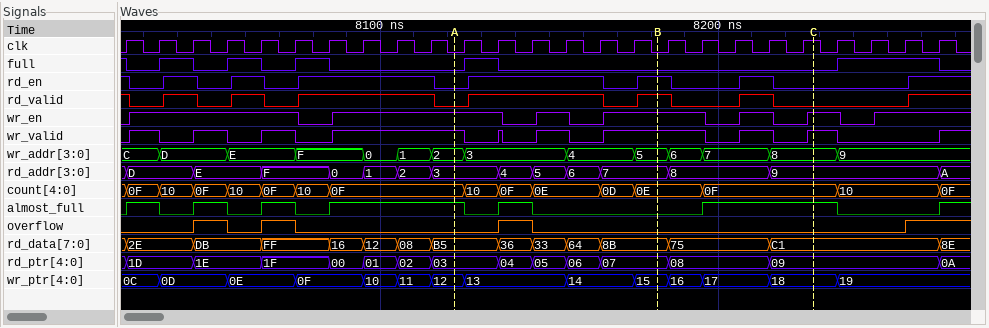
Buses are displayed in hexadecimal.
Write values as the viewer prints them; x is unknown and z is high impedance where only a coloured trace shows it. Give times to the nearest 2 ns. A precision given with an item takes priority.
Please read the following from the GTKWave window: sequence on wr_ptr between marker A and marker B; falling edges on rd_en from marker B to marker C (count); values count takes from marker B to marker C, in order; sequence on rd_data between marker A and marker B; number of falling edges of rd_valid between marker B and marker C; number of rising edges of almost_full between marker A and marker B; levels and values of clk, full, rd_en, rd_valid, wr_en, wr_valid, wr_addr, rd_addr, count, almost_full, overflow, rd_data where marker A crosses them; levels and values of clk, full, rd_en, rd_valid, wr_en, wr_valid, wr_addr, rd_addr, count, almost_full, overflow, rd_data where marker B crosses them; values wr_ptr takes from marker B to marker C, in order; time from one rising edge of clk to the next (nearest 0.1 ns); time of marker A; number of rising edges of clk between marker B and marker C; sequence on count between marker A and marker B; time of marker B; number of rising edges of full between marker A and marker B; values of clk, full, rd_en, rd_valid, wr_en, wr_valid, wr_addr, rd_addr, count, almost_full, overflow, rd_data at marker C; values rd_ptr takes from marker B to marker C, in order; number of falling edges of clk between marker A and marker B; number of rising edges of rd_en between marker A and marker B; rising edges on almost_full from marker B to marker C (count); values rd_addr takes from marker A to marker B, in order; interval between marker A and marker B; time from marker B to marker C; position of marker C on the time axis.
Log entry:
12, 13, 14, 15
2
0E, 0F
B5, 36, 33, 64, 8B
2
1
clk=0, full=0, rd_en=0, rd_valid=0, wr_en=1, wr_valid=1, wr_addr=2, rd_addr=3, count=0F, almost_full=1, overflow=0, rd_data=B5
clk=0, full=0, rd_en=1, rd_valid=1, wr_en=1, wr_valid=1, wr_addr=5, rd_addr=7, count=0E, almost_full=0, overflow=0, rd_data=8B
15, 16, 17, 18
10 ns
8122 ns
5
0F, 10, 0F, 0E, 0D, 0E
8182 ns
1
clk=1, full=0, rd_en=0, rd_valid=0, wr_en=1, wr_valid=1, wr_addr=8, rd_addr=9, count=0F, almost_full=1, overflow=0, rd_data=C1
07, 08, 09
6
2
1
3, 4, 5, 6, 7
60 ns
46 ns
8228 ns
